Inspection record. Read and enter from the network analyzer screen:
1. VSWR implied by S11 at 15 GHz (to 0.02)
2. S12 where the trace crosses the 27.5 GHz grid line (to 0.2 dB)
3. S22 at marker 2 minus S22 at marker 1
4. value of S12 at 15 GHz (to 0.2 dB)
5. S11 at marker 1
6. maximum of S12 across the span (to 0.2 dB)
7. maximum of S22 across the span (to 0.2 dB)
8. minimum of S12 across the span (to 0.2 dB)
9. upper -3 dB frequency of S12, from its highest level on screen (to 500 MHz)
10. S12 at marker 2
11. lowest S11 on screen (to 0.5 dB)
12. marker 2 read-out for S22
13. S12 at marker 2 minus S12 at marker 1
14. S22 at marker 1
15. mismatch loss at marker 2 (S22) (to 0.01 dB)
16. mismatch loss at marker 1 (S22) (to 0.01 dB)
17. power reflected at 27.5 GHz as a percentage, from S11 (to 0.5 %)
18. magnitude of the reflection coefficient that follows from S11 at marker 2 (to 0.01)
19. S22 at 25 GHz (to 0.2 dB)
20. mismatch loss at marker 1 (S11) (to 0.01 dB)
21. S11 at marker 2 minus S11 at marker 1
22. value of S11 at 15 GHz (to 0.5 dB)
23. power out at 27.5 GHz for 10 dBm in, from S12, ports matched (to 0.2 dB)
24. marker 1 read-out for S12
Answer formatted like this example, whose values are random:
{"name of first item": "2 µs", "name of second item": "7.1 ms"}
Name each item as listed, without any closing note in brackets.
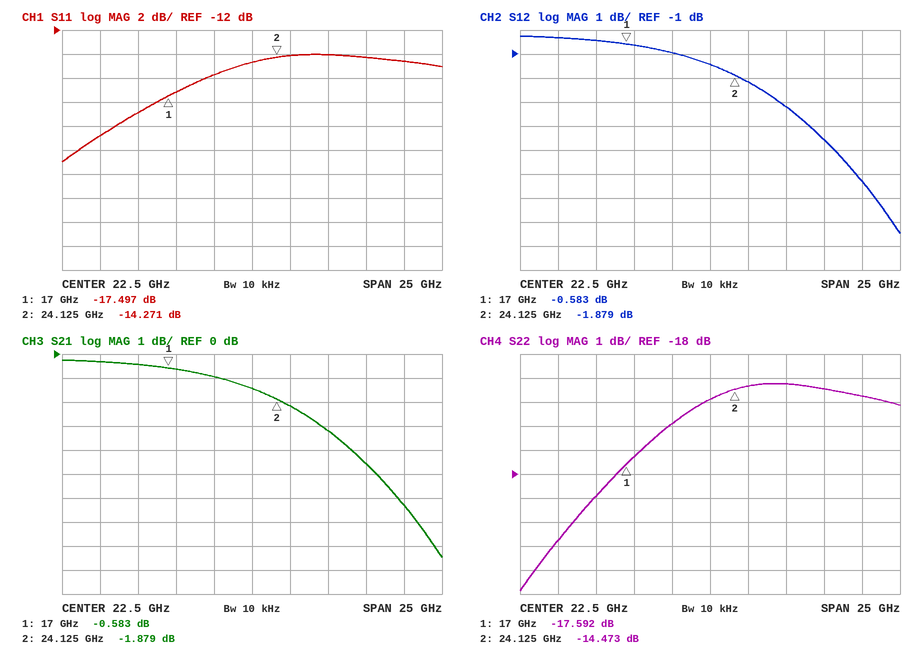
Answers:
{"VSWR implied by S11 at 15 GHz": "1.26", "S12 where the trace crosses the 27.5 GHz grid line": "-3.2 dB", "S22 at marker 2 minus S22 at marker 1": "3.119 dB", "value of S12 at 15 GHz": "-0.4 dB", "S11 at marker 1": "-17.497 dB", "maximum of S12 across the span": "-0.2 dB", "maximum of S22 across the span": "-14.2 dB", "minimum of S12 across the span": "-8.4 dB", "upper -3 dB frequency of S12, from its highest level on screen": "27.5 GHz", "S12 at marker 2": "-1.879 dB", "lowest S11 on screen": "-23.0 dB", "marker 2 read-out for S22": "-14.473 dB", "S12 at marker 2 minus S12 at marker 1": "-1.296 dB", "S22 at marker 1": "-17.592 dB", "mismatch loss at marker 2 (S22)": "0.16 dB", "mismatch loss at marker 1 (S22)": "0.08 dB", "power reflected at 27.5 GHz as a percentage, from S11": "4.0 %", "magnitude of the reflection coefficient that follows from S11 at marker 2": "0.19", "S22 at 25 GHz": "-14.4 dB", "mismatch loss at marker 1 (S11)": "0.08 dB", "S11 at marker 2 minus S11 at marker 1": "3.226 dB", "value of S11 at 15 GHz": "-19.0 dB", "power out at 27.5 GHz for 10 dBm in, from S12, ports matched": "6.8 dBm", "marker 1 read-out for S12": "-0.583 dB"}
